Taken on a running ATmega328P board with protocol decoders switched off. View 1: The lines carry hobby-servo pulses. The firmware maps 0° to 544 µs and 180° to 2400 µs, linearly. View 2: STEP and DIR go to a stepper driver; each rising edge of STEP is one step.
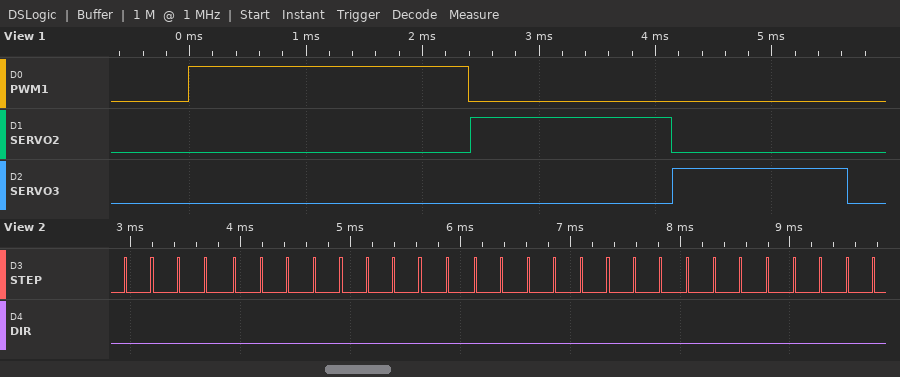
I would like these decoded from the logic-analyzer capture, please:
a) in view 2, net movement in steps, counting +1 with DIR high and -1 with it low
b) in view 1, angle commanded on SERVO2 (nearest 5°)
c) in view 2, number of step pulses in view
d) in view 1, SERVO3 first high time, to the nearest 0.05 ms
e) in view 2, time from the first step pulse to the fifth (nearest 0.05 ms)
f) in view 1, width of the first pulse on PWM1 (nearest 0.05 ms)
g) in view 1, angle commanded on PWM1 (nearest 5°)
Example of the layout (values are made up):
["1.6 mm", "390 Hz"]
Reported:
["-29", "115°", "29", "1.50 ms", "1.00 ms", "2.40 ms", "180°"]
